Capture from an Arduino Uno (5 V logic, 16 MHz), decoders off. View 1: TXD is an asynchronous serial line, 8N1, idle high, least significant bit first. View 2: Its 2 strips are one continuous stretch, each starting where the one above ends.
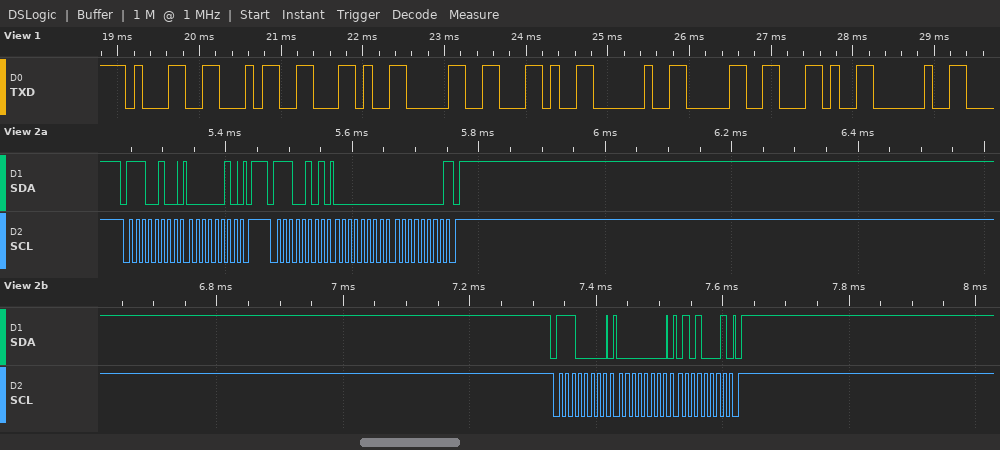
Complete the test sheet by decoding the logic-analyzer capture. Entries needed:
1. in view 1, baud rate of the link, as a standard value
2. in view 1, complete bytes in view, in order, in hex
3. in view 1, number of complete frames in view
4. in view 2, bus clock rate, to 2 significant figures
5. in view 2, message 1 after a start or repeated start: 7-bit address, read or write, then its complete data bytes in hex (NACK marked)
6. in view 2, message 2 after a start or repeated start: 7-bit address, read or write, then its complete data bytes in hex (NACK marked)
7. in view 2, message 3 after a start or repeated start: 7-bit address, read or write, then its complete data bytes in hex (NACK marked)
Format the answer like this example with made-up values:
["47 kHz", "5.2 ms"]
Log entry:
["9600 baud", "31 34 2C 30 2C 20 30 2C 20", "9", "100 kHz", "0x72 write: 02", "0x72 read: 00 00 NACK", "0x70 write: 00 51"]
